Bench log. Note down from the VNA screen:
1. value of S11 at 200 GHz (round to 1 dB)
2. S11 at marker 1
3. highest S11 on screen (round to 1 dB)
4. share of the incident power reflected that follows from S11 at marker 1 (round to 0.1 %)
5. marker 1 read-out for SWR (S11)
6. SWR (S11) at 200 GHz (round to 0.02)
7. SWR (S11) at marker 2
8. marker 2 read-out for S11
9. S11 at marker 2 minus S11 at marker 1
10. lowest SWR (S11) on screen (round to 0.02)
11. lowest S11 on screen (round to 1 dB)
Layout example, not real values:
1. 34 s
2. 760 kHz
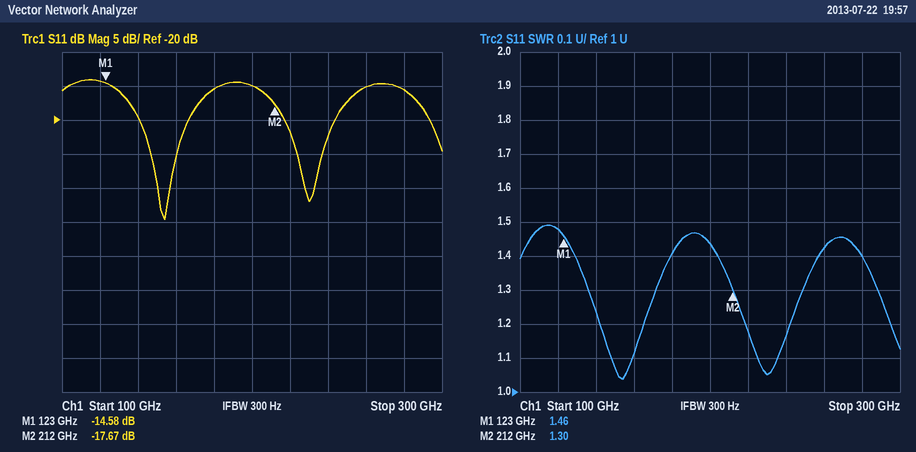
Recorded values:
1. -15 dB
2. -14.58 dB
3. -14 dB
4. 3.5 %
5. 1.46
6. 1.44
7. 1.30
8. -17.67 dB
9. -3.09 dB
10. 1.04
11. -35 dB
